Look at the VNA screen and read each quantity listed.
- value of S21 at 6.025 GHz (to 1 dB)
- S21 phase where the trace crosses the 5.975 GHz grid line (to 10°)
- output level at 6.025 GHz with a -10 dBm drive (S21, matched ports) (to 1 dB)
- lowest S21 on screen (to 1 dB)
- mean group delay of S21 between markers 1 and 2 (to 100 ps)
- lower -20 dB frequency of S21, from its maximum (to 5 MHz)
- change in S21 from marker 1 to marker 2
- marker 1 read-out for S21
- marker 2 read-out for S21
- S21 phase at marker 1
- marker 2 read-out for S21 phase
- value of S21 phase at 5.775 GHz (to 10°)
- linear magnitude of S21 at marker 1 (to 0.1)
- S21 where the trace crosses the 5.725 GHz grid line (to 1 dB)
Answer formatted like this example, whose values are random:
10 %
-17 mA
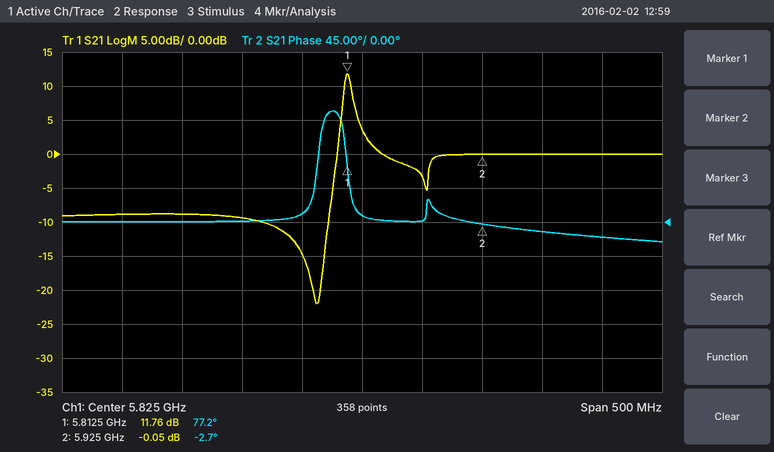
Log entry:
0 dB
-10°
-10 dBm
-22 dB
2.0 ns
5.800 GHz
-11.81 dB
11.76 dB
-0.05 dB
77.2°
-2.7°
10°
3.9
-9 dB
